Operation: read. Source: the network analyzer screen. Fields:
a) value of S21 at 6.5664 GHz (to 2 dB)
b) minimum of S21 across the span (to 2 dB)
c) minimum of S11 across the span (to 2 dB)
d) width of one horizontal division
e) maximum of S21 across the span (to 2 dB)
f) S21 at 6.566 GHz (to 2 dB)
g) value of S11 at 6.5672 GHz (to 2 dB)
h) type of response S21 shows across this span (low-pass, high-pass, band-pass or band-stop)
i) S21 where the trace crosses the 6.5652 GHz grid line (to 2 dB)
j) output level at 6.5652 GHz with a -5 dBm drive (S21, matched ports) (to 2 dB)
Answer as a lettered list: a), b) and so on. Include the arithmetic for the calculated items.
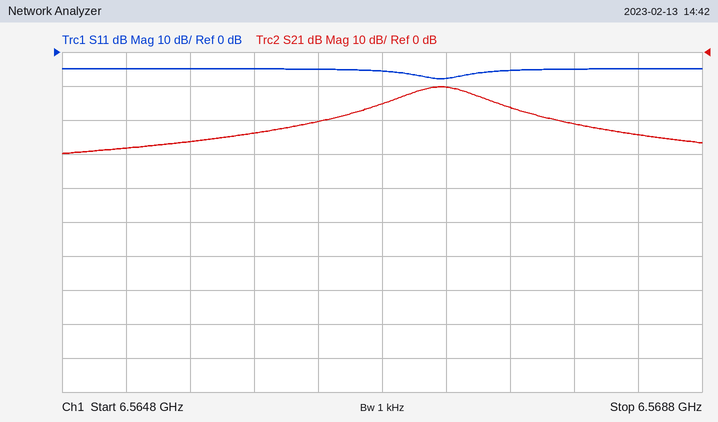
a) -20 dB
b) -30 dB
c) -8 dB
d) 400 kHz
e) -10 dB
f) -24 dB
g) -8 dB
h) band-pass
i) -28 dB
j) -5 dBm + (-28 dB) = -34 dBm
